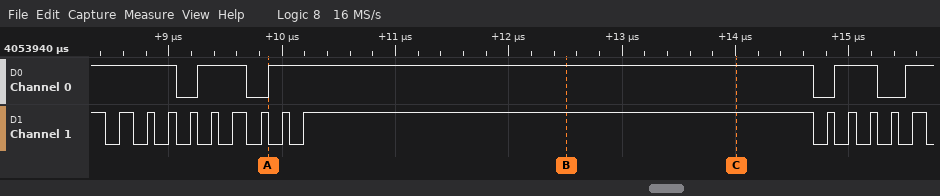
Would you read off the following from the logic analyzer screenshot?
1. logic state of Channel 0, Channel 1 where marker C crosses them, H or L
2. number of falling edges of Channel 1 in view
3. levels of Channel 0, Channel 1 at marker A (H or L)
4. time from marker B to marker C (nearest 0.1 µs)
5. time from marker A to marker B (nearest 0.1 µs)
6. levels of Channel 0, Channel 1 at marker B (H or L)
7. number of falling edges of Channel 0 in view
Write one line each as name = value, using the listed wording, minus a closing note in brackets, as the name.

logic state of Channel 0, Channel 1 where marker C crosses them, H or L = Channel 0=H, Channel 1=H
number of falling edges of Channel 1 in view = 15
levels of Channel 0, Channel 1 at marker A = Channel 0=H, Channel 1=L
time from marker B to marker C = 1.5 µs
time from marker A to marker B = 2.6 µs
levels of Channel 0, Channel 1 at marker B = Channel 0=H, Channel 1=H
number of falling edges of Channel 0 in view = 4
